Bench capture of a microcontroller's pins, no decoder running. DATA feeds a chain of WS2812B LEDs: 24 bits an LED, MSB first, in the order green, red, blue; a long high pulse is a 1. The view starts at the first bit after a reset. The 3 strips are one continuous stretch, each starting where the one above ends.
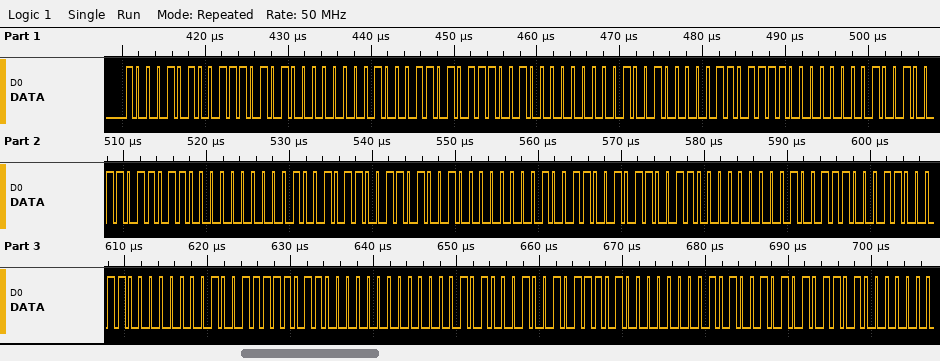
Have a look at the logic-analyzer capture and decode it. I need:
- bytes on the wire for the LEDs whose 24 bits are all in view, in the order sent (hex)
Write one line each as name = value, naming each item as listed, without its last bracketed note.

bytes on the wire for the LEDs whose 24 bits are all in view, in the order sent = 8A 75 00 8D 72 00 90 6F 00 93 6C 00 96 69 00 99 66 00 9C 63 00 9F 60 00 A2 5D 00
